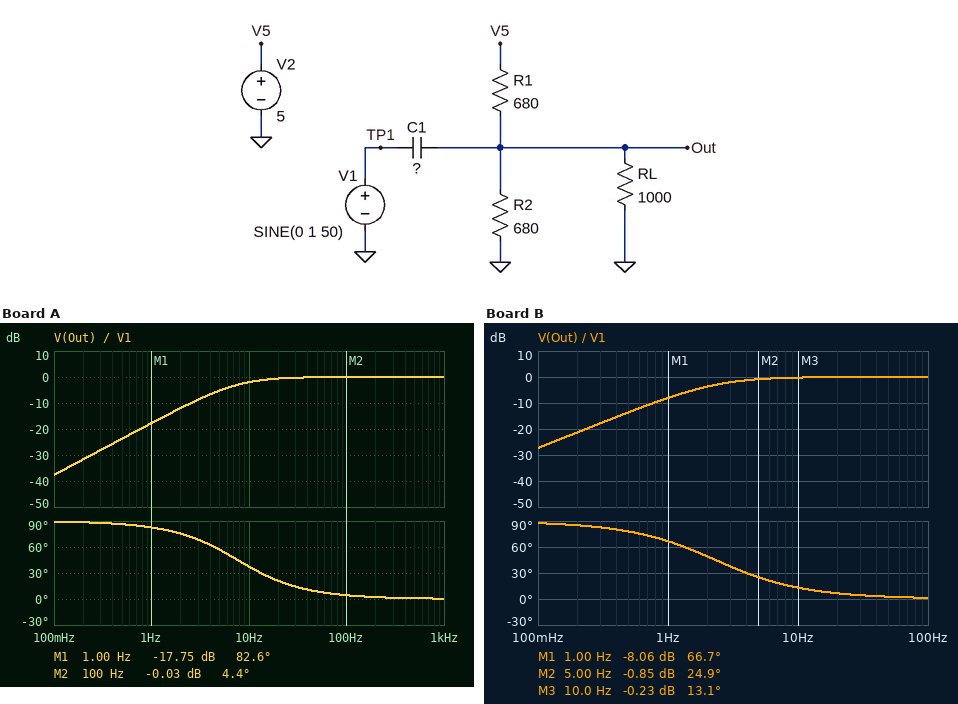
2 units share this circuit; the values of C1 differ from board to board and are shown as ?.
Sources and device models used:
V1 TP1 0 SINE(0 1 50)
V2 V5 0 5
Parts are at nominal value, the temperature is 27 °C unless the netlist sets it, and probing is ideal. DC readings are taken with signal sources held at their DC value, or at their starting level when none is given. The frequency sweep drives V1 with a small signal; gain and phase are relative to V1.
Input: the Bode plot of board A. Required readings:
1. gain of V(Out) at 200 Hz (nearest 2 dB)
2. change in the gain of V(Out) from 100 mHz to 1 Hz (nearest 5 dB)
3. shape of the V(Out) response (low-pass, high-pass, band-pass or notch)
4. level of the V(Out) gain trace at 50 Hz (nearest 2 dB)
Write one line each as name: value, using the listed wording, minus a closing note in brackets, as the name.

gain of V(Out) at 200 Hz: 0 dB
change in the gain of V(Out) from 100 mHz to 1 Hz: 20 dB
shape of the V(Out) response: high-pass
level of the V(Out) gain trace at 50 Hz: 0 dB
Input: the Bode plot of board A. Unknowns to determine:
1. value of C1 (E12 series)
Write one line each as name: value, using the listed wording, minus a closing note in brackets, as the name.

value of C1: 82 µF
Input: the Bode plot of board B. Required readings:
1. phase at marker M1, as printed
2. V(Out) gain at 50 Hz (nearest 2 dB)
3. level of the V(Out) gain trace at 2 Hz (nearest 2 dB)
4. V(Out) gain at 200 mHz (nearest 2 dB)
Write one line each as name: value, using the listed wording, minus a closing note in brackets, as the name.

phase at marker M1, as printed: 66.7 deg
V(Out) gain at 50 Hz: 0 dB
level of the V(Out) gain trace at 2 Hz: -4 dB
V(Out) gain at 200 mHz: -22 dB
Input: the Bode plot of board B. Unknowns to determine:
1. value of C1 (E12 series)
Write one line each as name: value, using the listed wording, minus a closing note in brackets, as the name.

value of C1: 270 µF
